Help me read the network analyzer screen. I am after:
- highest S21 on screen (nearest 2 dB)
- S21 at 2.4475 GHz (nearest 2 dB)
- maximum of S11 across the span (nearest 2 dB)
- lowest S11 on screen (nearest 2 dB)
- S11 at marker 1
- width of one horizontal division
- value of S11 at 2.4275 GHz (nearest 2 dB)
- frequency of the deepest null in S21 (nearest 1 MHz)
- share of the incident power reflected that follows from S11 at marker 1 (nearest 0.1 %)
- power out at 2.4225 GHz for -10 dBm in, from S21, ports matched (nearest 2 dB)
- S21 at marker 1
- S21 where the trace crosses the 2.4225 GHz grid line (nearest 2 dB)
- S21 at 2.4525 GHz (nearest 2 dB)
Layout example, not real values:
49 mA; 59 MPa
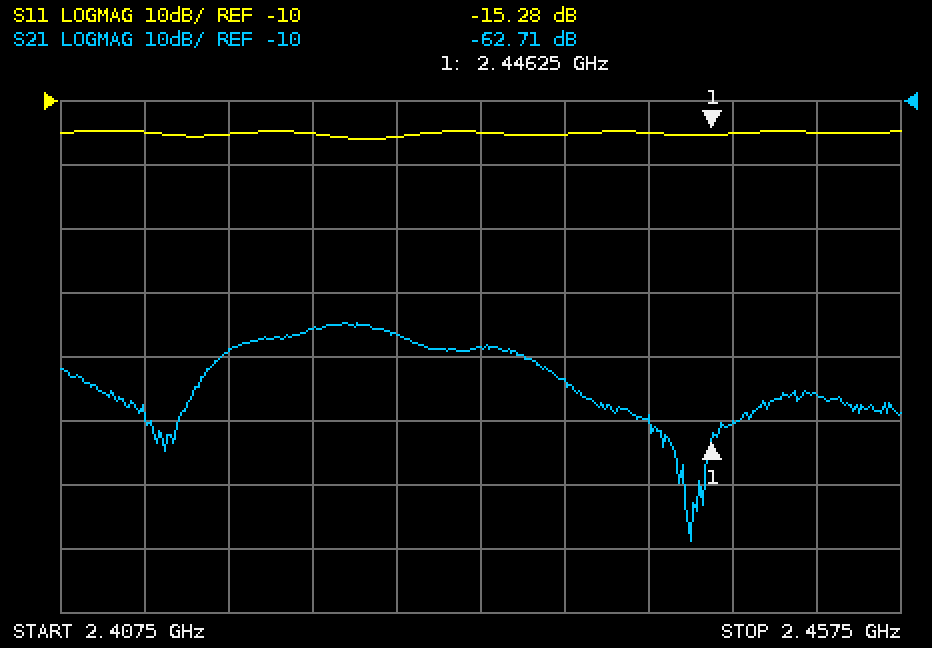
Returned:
-44 dB; -60 dB; -14 dB; -16 dB; -15.28 dB; 5 MHz; -16 dB; 2.445 GHz; 3.0 %; -56 dBm; -62.71 dB; -46 dB; -56 dB
